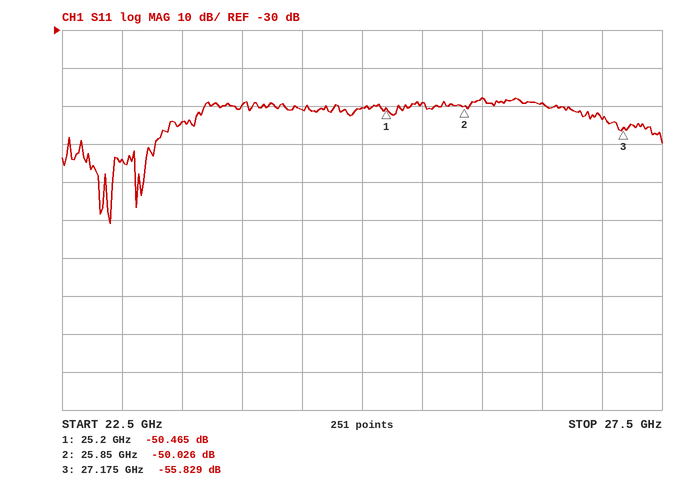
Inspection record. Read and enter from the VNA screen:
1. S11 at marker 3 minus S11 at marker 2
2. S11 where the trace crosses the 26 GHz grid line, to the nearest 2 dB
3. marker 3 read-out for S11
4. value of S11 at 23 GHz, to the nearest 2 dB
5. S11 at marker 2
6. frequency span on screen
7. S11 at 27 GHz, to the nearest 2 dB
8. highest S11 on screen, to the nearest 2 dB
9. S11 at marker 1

-5.803 dB
-48 dB
-55.829 dB
-64 dB
-50.026 dB
5 GHz
-54 dB
-48 dB
-50.465 dB
